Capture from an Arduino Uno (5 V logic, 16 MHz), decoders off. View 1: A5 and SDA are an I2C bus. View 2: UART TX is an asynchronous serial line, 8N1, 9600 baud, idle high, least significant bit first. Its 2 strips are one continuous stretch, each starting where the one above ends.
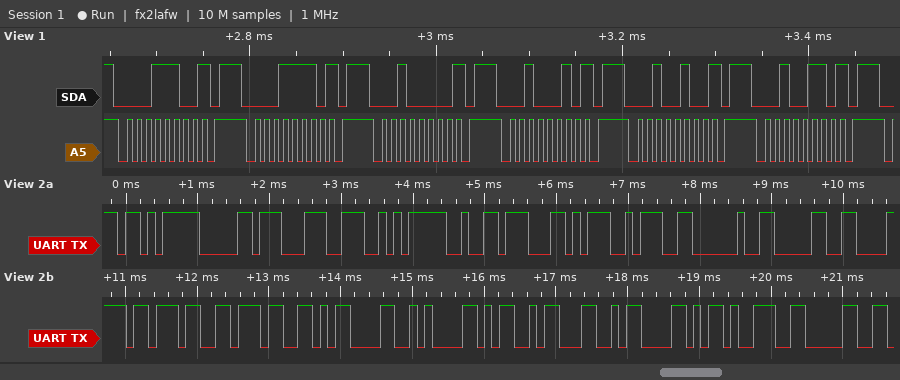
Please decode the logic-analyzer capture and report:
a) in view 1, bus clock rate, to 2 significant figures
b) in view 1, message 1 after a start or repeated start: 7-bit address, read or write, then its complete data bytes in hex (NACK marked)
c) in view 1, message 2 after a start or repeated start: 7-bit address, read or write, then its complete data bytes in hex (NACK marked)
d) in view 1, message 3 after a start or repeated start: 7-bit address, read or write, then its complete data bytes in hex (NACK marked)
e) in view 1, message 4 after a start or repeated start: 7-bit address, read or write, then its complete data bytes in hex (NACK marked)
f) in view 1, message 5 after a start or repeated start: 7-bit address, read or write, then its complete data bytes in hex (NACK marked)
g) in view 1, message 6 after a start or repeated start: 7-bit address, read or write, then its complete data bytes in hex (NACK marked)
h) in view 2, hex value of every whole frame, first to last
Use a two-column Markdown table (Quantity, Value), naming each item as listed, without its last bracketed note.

| Quantity | Value |
|---|---|
| in view 1, bus clock rate, to 2 significant figures | 100 kHz |
| in view 1, message 1 after a start or repeated start: 7-bit address, read or write, then its complete data bytes in hex | 0x0E write NACK |
| in view 1, message 2 after a start or repeated start: 7-bit address, read or write, then its complete data bytes in hex | 0x0F write NACK |
| in view 1, message 3 after a start or repeated start: 7-bit address, read or write, then its complete data bytes in hex | 0x10 write NACK |
| in view 1, message 4 after a start or repeated start: 7-bit address, read or write, then its complete data bytes in hex | 0x11 write NACK |
| in view 1, message 5 after a start or repeated start: 7-bit address, read or write, then its complete data bytes in hex | 0x12 write NACK |
| in view 1, message 6 after a start or repeated start: 7-bit address, read or write, then its complete data bytes in hex | 0x13 write NACK |
| in view 2, hex value of every whole frame, first to last | EB B0 9C EA B2 AC 3A 20 30 78 37 37 0D 0A 4D 4C 58 39 30 |
